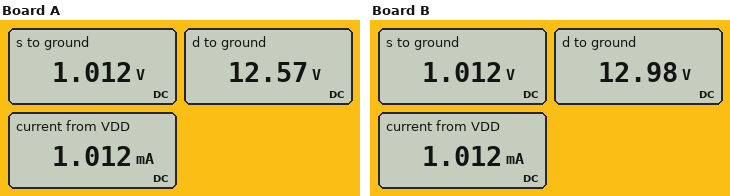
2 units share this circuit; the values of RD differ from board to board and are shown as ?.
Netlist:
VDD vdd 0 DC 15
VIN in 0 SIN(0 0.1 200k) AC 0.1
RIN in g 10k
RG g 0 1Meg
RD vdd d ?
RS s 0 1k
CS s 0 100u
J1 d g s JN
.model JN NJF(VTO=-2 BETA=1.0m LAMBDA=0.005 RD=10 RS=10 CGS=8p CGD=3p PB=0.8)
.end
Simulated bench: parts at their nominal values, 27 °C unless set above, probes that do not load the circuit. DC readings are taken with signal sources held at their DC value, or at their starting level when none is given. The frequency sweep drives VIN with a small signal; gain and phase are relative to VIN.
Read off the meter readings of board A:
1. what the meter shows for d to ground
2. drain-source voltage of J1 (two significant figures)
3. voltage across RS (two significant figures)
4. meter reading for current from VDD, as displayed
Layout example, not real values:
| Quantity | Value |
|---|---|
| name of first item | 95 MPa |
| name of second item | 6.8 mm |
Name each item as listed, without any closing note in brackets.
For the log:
| Quantity | Value |
|---|---|
| what the meter shows for d to ground | 12.57 V |
| drain-source voltage of J1 | 12 V |
| voltage across RS | 1.0 V |
| meter reading for current from VDD, as displayed | 1.012 mA |
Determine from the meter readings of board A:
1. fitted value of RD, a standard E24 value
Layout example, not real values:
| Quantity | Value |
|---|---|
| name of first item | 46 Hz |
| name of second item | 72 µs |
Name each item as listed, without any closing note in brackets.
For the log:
| Quantity | Value |
|---|---|
| fitted value of RD, a standard E24 value | 2.4 kΩ |
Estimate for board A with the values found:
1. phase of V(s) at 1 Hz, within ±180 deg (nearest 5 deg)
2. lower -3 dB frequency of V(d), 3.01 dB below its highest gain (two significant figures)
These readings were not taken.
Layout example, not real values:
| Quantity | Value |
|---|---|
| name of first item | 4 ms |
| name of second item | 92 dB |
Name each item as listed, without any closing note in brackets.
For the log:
| Quantity | Value |
|---|---|
| phase of V(s) at 1 Hz, within ±180 deg | -10 deg |
| lower -3 dB frequency of V(d), 3.01 dB below its highest gain | 4.2 Hz |
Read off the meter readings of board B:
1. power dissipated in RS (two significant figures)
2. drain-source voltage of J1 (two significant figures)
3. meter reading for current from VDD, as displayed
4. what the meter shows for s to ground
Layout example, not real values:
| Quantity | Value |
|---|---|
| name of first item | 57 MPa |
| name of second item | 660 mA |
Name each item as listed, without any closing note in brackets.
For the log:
| Quantity | Value |
|---|---|
| power dissipated in RS | 1.0 mW |
| drain-source voltage of J1 | 12 V |
| meter reading for current from VDD, as displayed | 1.012 mA |
| what the meter shows for s to ground | 1.012 V |
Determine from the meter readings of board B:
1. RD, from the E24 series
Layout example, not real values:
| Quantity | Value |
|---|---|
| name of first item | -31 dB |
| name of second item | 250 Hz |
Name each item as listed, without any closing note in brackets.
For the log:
| Quantity | Value |
|---|---|
| RD, from the E24 series | 2 kΩ |
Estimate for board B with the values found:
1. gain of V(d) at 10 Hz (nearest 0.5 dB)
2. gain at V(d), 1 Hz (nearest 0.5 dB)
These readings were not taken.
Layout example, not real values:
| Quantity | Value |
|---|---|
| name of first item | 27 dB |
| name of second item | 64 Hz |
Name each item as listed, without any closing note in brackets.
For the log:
| Quantity | Value |
|---|---|
| gain of V(d) at 10 Hz | 11.0 dB |
| gain at V(d), 1 Hz | 3.5 dB |
